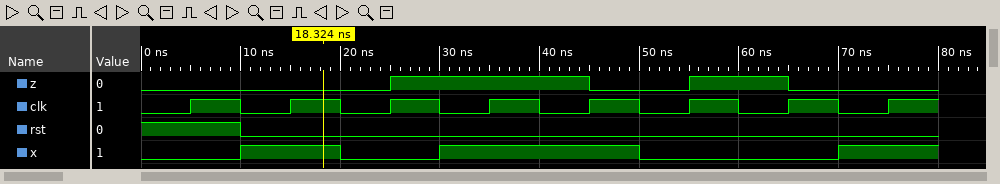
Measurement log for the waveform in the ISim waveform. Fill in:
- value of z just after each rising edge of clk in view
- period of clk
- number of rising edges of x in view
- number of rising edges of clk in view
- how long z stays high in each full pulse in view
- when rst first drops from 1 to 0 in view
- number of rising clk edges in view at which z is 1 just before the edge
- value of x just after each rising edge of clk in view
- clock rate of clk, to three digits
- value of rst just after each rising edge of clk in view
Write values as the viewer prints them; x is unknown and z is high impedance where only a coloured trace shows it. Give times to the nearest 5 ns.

0 0 1 1 0 1 0 0
10 ns
3
8
20 ns, 10 ns
10 ns
3
0 1 0 1 1 0 0 1
100 MHz
1 0 0 0 0 0 0 0
